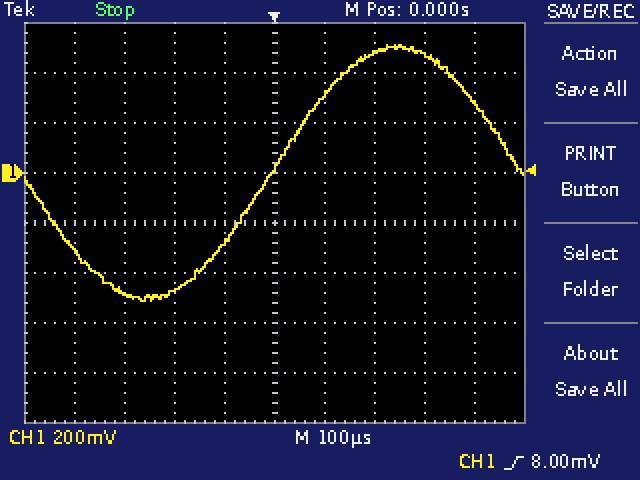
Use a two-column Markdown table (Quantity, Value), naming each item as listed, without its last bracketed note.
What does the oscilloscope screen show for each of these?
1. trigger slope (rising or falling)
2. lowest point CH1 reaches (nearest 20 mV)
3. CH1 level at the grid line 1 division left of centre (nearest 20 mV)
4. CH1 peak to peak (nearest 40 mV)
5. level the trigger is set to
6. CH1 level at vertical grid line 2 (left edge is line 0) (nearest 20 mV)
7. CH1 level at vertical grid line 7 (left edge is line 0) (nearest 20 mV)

| Quantity | Value |
|---|---|
| trigger slope | rising |
| lowest point CH1 reaches | -520 mV |
| CH1 level at the grid line 1 division left of centre | -280 mV |
| CH1 peak to peak | 1.04 V |
| level the trigger is set to | 8.00 mV |
| CH1 level at vertical grid line 2 (left edge is line 0) | -480 mV |
| CH1 level at vertical grid line 7 (left edge is line 0) | 480 mV |
